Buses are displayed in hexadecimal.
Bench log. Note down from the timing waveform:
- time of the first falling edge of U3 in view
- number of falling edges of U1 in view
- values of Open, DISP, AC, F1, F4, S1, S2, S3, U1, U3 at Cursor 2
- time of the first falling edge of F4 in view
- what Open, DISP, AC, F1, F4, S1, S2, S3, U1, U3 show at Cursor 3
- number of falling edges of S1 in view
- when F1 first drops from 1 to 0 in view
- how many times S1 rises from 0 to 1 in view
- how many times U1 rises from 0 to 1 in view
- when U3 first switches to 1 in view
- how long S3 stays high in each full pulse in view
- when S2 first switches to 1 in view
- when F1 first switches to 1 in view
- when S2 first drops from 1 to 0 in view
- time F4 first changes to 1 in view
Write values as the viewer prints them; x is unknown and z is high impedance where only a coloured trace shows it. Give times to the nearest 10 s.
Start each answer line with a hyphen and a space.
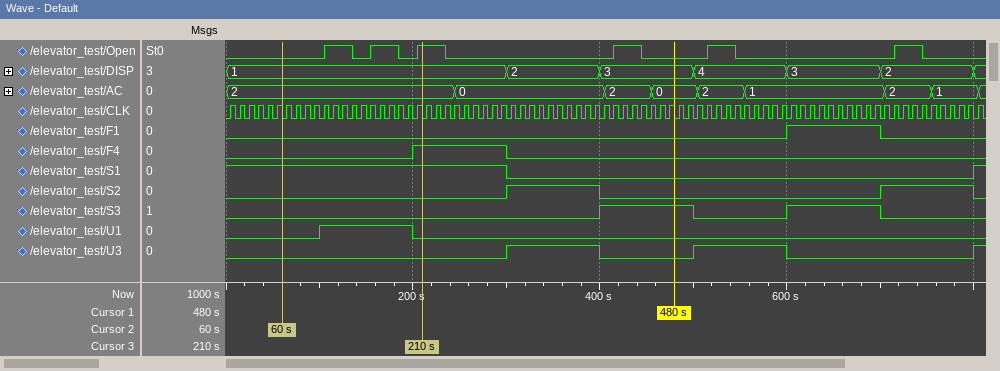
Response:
- 400 s
- 1
- Open=0, DISP=1, AC=2, F1=0, F4=0, S1=1, S2=0, S3=0, U1=0, U3=0
- 300 s
- Open=1, DISP=1, AC=2, F1=0, F4=1, S1=1, S2=0, S3=0, U1=0, U3=0
- 1
- 700 s
- 1
- 1
- 300 s
- 100 s, 100 s
- 300 s
- 600 s
- 400 s
- 200 s
